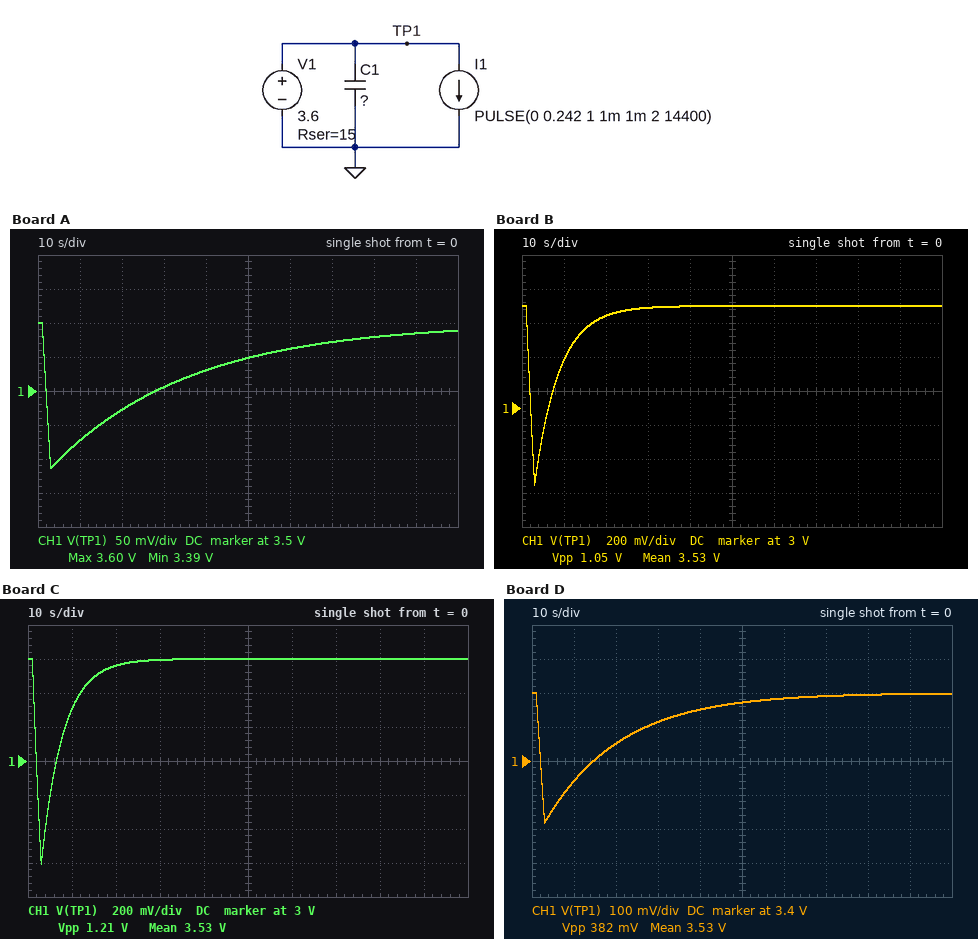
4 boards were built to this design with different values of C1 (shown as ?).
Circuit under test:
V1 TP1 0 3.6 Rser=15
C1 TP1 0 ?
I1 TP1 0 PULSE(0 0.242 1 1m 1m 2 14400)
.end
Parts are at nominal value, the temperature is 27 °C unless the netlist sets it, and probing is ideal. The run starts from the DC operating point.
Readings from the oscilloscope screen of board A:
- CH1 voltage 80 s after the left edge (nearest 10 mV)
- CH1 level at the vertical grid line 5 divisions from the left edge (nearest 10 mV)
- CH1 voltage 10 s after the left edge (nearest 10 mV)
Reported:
3.58 V
3.55 V
3.43 V
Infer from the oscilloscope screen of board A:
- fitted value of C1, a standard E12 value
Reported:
2.2 F
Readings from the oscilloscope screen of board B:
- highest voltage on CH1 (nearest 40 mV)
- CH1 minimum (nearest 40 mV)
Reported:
3.60 V
2.56 V
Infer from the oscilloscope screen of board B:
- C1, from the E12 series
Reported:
390 mF
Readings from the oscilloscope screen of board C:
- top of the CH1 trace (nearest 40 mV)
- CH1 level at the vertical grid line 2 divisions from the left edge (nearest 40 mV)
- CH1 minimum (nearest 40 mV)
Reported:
3.60 V
3.56 V
2.40 V
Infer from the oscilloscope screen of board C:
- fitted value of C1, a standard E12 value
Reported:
330 mF
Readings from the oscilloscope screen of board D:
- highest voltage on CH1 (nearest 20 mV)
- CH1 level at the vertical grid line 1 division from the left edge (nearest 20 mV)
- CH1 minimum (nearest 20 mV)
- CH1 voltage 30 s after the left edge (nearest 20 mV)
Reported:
3.60 V
3.34 V
3.22 V
3.52 V
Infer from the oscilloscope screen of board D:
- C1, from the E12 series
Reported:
1.2 F
